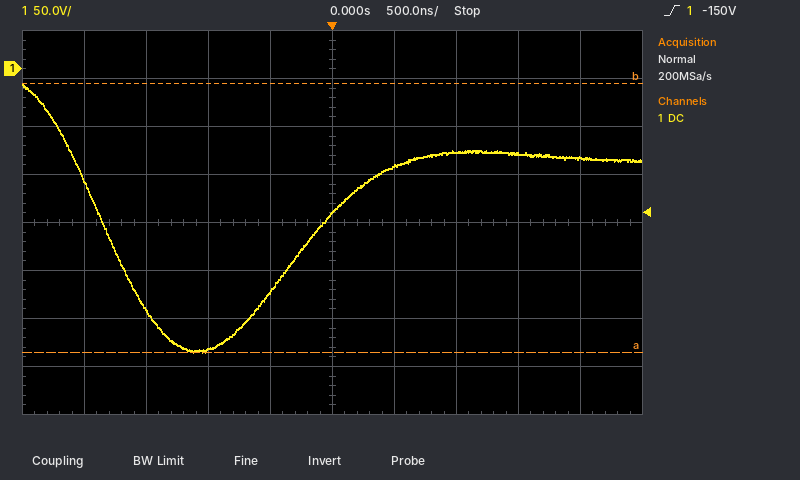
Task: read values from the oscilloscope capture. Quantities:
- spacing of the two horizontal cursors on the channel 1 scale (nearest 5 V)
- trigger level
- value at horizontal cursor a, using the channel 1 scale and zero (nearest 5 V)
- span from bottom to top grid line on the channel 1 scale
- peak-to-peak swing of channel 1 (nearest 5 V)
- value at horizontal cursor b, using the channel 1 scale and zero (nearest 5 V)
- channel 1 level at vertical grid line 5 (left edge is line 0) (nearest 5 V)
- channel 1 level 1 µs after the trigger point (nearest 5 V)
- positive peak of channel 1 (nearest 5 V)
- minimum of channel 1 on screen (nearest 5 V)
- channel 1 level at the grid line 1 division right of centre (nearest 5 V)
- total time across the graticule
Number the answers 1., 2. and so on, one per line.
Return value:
1. 280 V
2. -150 V
3. -295 V
4. 400 V
5. 280 V
6. -15 V
7. -150 V
8. -85 V
9. -15 V
10. -295 V
11. -100 V
12. 5 µs
